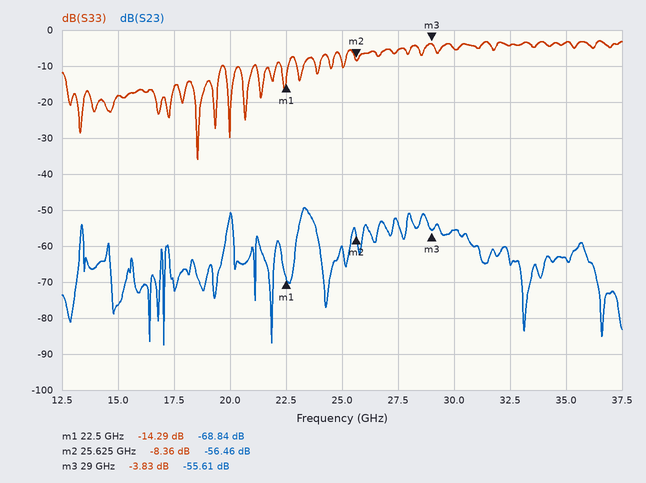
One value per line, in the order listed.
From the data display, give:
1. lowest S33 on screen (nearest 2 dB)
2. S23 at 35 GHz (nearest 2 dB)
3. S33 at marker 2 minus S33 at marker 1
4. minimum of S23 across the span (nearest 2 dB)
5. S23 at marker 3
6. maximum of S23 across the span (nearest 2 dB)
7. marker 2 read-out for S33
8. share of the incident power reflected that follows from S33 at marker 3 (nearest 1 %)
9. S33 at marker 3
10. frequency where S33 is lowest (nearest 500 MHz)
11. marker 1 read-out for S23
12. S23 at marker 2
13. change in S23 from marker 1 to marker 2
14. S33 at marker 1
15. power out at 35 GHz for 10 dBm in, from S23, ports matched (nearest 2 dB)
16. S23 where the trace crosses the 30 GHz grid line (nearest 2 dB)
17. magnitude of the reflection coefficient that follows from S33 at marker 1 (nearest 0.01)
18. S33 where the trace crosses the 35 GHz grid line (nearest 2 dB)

-36 dB
-64 dB
5.93 dB
-88 dB
-55.61 dB
-50 dB
-8.36 dB
41 %
-3.83 dB
18.5 GHz
-68.84 dB
-56.46 dB
12.38 dB
-14.29 dB
-54 dBm
-56 dB
0.19
-4 dB
